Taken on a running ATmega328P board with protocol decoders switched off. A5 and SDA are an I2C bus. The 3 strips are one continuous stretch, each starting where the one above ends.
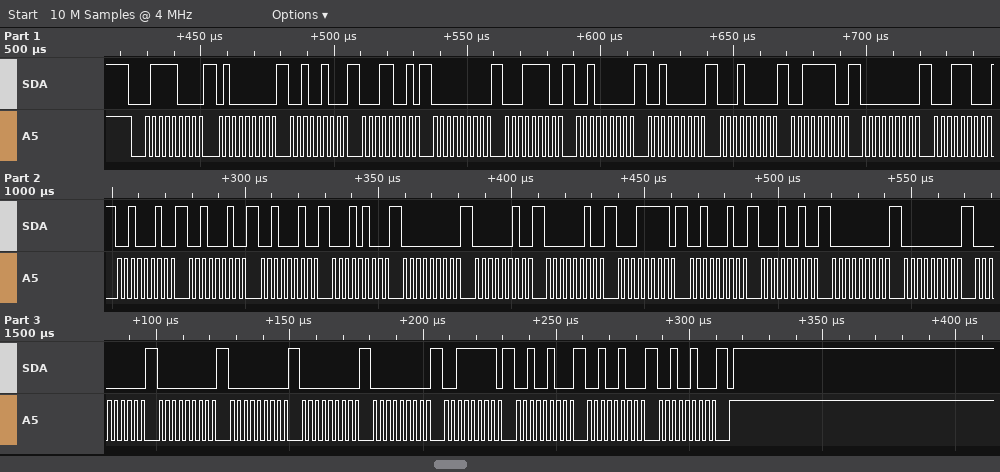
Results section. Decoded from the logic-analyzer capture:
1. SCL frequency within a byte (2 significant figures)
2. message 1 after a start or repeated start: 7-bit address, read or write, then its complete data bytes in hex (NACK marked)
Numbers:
400 kHz
0x3C write: 40 24 19 00 1E 20 20 10 3E 00 1C 22 22 22 14 00 02 02 1F 22 12 00 00 00 00 00 00 00 3F 24 24 24
